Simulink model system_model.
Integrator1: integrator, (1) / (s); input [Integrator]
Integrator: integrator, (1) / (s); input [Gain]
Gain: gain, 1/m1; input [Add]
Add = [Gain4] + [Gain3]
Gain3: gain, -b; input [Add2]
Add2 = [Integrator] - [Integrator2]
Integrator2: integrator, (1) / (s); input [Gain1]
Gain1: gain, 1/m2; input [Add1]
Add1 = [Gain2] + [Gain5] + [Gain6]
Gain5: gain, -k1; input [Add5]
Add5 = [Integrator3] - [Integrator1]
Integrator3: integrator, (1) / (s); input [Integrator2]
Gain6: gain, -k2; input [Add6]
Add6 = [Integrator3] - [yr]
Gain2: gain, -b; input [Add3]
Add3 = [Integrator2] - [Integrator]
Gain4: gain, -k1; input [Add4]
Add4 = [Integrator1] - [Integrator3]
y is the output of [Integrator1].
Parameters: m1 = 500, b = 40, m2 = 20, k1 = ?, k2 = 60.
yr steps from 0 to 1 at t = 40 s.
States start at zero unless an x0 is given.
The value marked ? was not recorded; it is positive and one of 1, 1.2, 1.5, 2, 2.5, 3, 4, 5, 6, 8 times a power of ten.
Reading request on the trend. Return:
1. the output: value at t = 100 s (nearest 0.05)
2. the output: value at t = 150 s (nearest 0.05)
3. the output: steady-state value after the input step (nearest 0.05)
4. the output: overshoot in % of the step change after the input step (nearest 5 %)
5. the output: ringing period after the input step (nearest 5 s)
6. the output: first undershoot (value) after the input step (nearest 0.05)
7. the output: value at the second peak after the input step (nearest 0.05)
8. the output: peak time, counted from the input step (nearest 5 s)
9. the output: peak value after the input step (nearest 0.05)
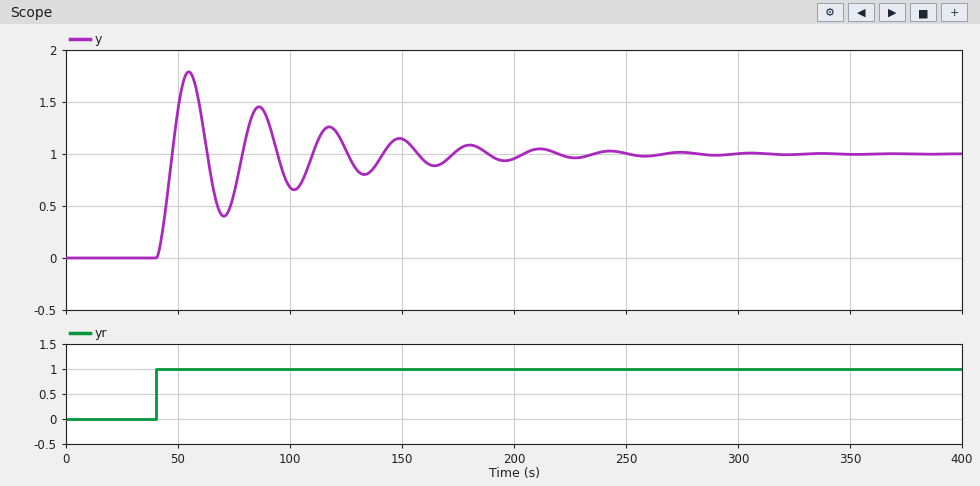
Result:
0.70
1.15
1.00
80 %
30 s
0.40
1.45
15 s
1.80
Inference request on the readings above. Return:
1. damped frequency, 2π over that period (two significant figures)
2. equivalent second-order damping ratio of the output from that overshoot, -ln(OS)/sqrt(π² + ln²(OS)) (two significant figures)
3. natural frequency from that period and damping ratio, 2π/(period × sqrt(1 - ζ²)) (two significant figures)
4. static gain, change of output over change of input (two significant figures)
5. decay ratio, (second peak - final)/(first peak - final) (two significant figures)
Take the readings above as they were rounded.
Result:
0.21 rad/s
0.071
0.21 rad/s
1.0
0.56
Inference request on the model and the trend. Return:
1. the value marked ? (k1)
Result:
30
